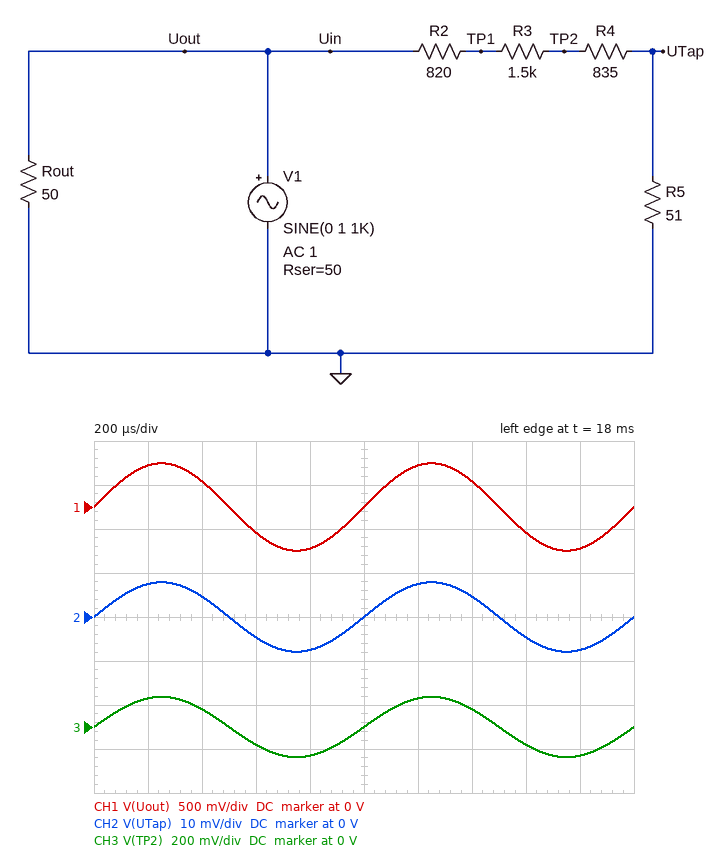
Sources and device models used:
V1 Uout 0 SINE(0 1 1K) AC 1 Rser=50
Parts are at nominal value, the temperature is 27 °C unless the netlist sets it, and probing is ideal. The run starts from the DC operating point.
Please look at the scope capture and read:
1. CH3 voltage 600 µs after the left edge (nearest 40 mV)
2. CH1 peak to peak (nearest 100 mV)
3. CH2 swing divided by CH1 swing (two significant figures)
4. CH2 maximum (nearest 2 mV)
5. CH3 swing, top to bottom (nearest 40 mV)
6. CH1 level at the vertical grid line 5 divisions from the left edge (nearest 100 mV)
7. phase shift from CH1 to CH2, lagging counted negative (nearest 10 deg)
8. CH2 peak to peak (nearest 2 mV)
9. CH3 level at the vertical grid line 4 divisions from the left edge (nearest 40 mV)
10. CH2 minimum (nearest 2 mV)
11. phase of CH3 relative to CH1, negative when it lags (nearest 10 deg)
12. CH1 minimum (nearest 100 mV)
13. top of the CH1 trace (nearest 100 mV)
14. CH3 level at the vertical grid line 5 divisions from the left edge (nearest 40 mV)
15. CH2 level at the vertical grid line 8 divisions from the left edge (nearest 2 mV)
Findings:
-80 mV
1.0 V
0.016
8 mV
280 mV
0 V
0 deg
16 mV
-120 mV
-8 mV
0 deg
-500 mV
500 mV
0 V
-4 mV
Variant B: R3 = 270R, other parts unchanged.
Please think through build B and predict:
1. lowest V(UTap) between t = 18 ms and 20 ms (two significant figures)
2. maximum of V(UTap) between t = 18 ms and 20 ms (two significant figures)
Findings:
-13 mV
13 mV
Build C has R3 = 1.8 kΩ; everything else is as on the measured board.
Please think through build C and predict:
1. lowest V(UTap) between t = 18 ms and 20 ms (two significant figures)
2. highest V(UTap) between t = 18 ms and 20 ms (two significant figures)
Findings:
-7.2 mV
7.2 mV
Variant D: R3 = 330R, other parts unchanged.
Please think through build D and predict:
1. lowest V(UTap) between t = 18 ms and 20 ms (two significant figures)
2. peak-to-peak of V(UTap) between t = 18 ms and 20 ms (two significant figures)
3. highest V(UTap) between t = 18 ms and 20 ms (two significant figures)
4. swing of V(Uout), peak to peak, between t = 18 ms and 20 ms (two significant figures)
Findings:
-12 mV
25 mV
12 mV
990 mV
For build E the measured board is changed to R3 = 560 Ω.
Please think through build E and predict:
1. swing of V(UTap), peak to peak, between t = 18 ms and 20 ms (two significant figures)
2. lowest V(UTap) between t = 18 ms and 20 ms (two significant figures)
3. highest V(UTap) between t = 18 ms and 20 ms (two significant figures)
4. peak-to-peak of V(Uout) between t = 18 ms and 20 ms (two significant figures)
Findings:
22 mV
-11 mV
11 mV
990 mV
